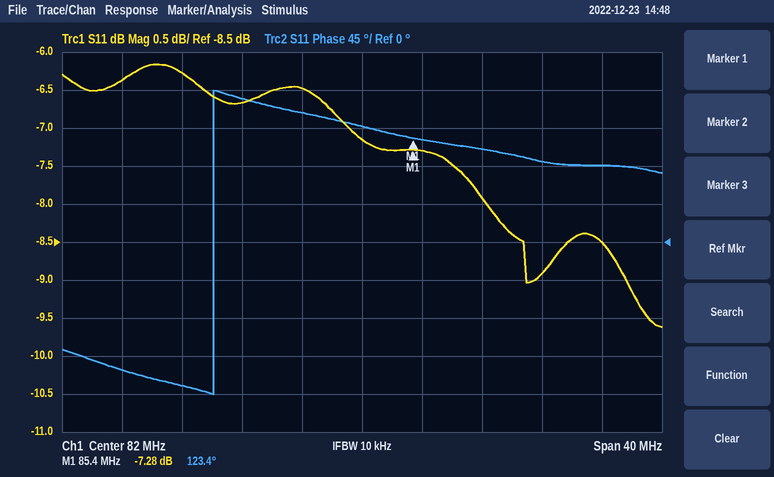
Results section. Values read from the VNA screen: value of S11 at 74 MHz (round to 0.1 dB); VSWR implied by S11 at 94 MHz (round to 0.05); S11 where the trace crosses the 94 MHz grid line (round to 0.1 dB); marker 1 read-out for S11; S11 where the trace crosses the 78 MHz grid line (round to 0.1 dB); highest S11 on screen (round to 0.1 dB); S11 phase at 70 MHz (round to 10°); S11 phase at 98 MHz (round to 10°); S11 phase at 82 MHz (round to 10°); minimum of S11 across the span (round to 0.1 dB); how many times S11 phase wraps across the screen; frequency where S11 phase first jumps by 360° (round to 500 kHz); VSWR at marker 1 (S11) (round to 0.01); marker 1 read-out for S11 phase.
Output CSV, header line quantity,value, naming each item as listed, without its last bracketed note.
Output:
quantity,value
value of S11 at 74 MHz,-6.7 dB
VSWR implied by S11 at 94 MHz,2.10
S11 where the trace crosses the 94 MHz grid line,-8.9 dB
marker 1 read-out for S11,-7.28 dB
S11 where the trace crosses the 78 MHz grid line,-6.5 dB
highest S11 on screen,-6.2 dB
S11 phase at 70 MHz,-170°
S11 phase at 98 MHz,90°
S11 phase at 82 MHz,140°
minimum of S11 across the span,-9.6 dB
how many times S11 phase wraps across the screen,1
frequency where S11 phase first jumps by 360°,72.0 MHz
VSWR at marker 1 (S11),2.52
marker 1 read-out for S11 phase,123.4°
